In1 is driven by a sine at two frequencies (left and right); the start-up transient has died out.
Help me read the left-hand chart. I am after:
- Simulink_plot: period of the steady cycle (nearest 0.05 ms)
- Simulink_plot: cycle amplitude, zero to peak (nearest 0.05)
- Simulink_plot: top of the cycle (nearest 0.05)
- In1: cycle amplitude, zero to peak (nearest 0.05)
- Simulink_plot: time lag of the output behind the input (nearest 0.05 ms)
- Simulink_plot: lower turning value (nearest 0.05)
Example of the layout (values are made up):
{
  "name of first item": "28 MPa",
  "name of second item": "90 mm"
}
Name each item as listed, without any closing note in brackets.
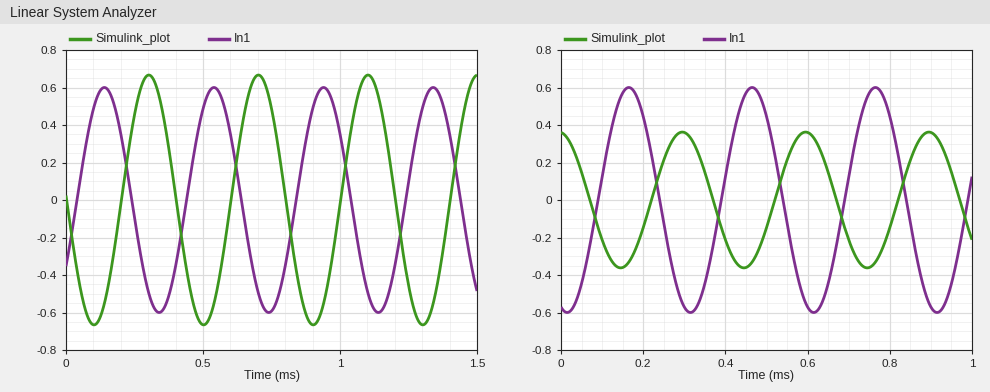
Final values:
{
  "Simulink_plot: period of the steady cycle": "0.40 ms",
  "Simulink_plot: cycle amplitude, zero to peak": "0.65",
  "Simulink_plot: top of the cycle": "0.65",
  "In1: cycle amplitude, zero to peak": "0.60",
  "Simulink_plot: time lag of the output behind the input": "0.15 ms",
  "Simulink_plot: lower turning value": "-0.65"
}
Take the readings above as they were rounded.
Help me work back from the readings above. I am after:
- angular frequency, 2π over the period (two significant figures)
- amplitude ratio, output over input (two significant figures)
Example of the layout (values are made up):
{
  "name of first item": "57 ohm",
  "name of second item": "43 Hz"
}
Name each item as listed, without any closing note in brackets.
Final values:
{
  "angular frequency, 2π over the period": "16 rad/ms",
  "amplitude ratio, output over input": "1.1"
}
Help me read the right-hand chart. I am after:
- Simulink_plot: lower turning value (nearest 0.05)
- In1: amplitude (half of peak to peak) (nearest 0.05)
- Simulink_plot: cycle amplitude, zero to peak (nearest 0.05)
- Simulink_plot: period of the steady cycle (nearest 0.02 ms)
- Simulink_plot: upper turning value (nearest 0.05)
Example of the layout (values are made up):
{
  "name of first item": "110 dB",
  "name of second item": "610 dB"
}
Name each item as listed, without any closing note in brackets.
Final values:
{
  "Simulink_plot: lower turning value": "-0.35",
  "In1: amplitude (half of peak to peak)": "0.60",
  "Simulink_plot: cycle amplitude, zero to peak": "0.35",
  "Simulink_plot: period of the steady cycle": "0.30 ms",
  "Simulink_plot: upper turning value": "0.35"
}
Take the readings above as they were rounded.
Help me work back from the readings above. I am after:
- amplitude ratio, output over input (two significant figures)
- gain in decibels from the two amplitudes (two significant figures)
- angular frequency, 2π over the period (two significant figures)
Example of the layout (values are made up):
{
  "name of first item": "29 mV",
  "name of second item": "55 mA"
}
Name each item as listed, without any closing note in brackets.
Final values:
{
  "amplitude ratio, output over input": "0.58",
  "gain in decibels from the two amplitudes": "-4.7 dB",
  "angular frequency, 2π over the period": "21 rad/ms"
}
